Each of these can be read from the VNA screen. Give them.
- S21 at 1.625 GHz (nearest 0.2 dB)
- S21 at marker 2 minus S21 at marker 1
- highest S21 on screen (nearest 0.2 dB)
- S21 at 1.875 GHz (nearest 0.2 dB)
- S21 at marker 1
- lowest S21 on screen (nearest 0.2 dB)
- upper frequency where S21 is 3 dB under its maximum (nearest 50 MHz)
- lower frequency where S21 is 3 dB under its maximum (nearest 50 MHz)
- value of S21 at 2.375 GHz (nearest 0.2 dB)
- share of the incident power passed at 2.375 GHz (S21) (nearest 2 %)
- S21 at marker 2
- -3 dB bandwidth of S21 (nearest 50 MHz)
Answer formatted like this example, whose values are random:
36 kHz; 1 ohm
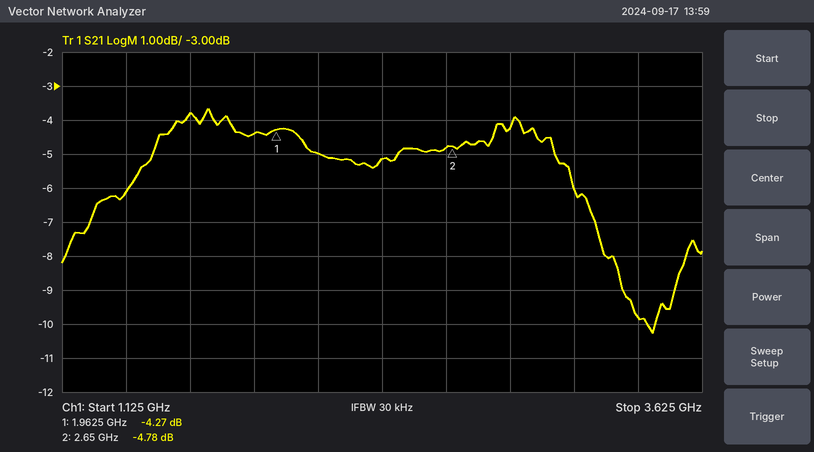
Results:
-3.8 dB; -0.51 dB; -3.6 dB; -4.4 dB; -4.27 dB; -10.2 dB; 3.20 GHz; 1.25 GHz; -5.2 dB; 30 %; -4.78 dB; 1.95 GHz
